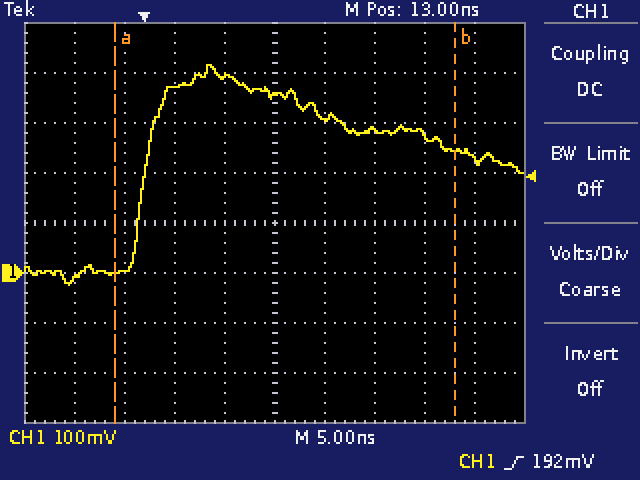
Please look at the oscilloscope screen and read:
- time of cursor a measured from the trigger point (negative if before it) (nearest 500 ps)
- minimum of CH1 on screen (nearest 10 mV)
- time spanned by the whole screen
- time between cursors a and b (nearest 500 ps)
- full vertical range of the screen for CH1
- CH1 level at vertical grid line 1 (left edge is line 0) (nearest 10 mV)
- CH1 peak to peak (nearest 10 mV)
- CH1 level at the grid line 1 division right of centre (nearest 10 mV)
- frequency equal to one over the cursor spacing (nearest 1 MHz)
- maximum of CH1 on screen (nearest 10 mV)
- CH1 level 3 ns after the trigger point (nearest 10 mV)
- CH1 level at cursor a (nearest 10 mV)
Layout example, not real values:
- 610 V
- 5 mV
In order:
- -3.0 ns
- -20 mV
- 50 ns
- 34.0 ns
- 800 mV
- -10 mV
- 440 mV
- 310 mV
- 29 MHz
- 420 mV
- 370 mV
- 0 mV
